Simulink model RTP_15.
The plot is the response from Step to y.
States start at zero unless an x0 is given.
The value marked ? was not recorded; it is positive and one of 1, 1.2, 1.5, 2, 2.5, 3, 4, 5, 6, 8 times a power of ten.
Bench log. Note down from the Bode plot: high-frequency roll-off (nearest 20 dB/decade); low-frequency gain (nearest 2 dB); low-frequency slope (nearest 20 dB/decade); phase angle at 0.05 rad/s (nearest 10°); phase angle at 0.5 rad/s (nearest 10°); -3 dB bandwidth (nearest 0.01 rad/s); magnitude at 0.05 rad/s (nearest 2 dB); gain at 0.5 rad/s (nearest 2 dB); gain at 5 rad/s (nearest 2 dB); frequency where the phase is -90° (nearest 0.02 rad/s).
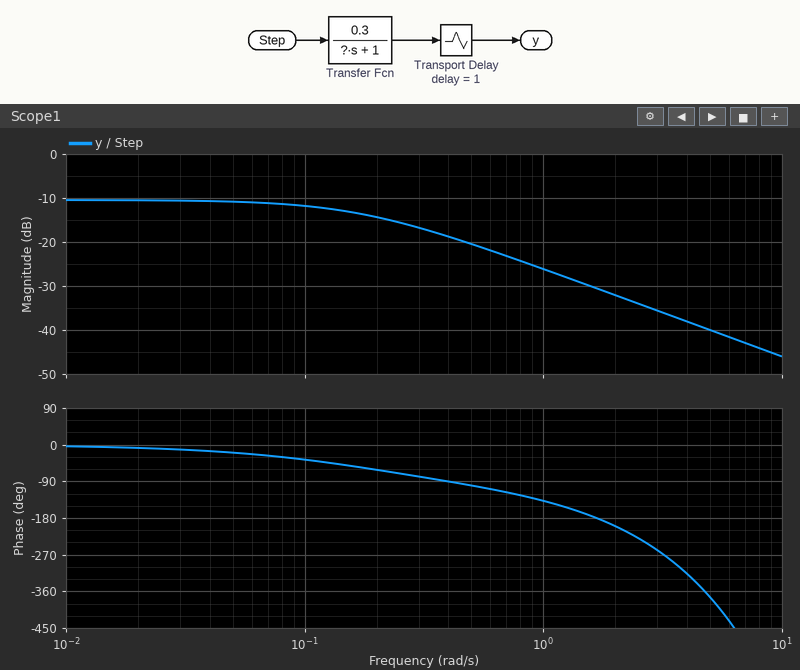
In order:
-20 dB/decade
-10 dB
0 dB/decade
-20°
-100°
0.17 rad/s
-10 dB
-20 dB
-40 dB
0.40 rad/s
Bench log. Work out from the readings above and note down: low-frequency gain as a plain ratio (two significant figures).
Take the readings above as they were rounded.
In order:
0.32
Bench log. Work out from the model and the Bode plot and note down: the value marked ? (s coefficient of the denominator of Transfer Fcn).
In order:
6
